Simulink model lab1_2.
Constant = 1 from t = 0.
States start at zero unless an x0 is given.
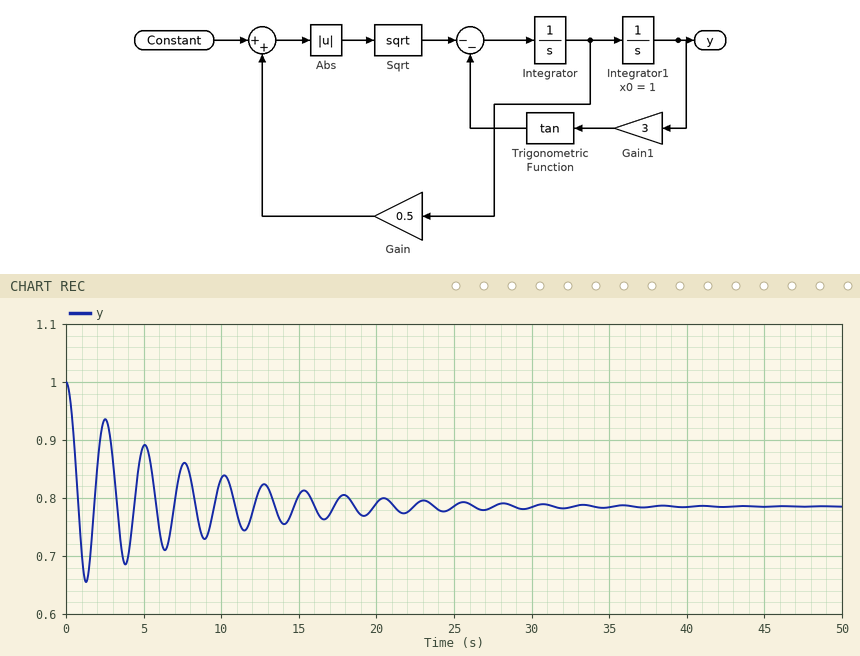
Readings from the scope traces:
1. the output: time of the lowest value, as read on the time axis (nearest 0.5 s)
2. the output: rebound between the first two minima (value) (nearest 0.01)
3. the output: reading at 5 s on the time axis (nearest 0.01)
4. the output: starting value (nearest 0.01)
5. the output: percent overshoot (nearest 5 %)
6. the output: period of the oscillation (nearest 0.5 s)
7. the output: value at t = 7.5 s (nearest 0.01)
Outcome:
1.5 s
0.94
0.89
1.00
60 %
2.5 s
0.86
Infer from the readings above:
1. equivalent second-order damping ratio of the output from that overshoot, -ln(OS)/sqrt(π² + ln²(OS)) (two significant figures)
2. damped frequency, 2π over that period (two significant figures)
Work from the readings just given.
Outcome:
0.16
2.5 rad/s
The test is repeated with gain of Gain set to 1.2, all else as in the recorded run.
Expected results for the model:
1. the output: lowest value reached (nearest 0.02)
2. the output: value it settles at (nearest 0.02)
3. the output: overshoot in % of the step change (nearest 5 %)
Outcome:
0.68
0.78
50 %
